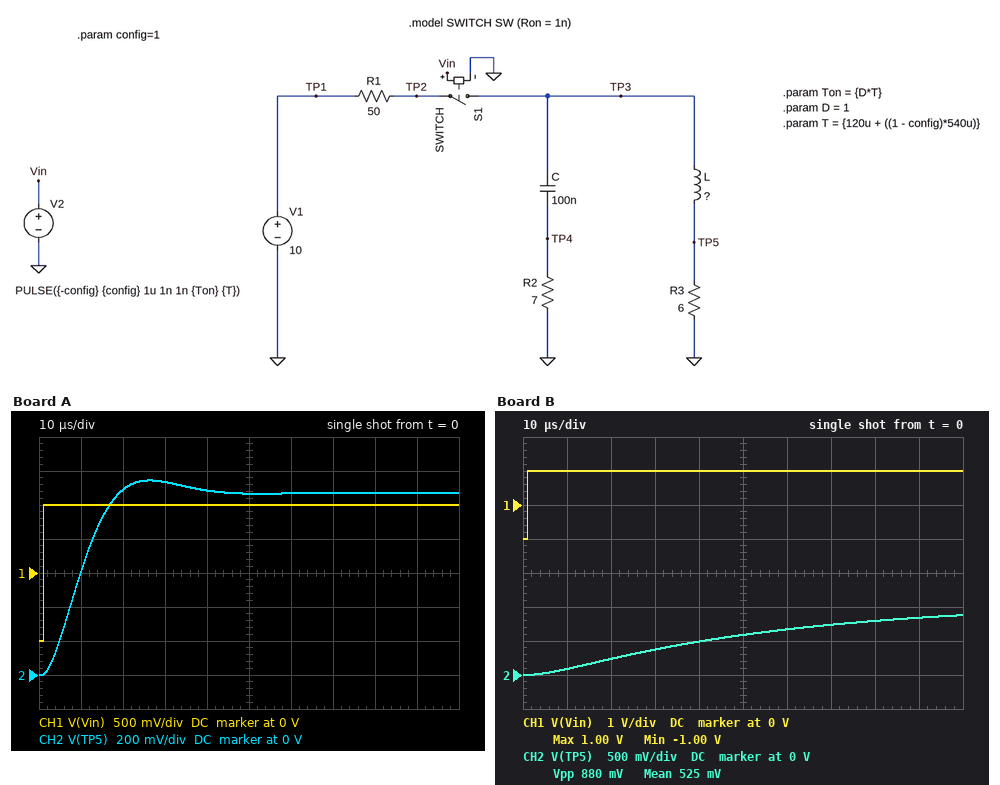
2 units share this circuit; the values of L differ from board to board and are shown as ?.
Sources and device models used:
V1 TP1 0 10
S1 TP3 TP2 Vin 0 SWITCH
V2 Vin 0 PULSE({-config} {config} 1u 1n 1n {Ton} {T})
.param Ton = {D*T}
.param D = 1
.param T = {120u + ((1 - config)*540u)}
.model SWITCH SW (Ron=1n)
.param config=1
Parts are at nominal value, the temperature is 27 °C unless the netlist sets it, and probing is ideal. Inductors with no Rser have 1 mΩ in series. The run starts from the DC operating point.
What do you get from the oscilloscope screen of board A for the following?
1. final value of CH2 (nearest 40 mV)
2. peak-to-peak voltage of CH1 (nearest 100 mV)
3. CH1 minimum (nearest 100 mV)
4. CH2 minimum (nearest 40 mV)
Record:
1.08 V
2.0 V
-1.0 V
0 V
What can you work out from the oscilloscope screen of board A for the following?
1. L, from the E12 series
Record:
390 µH
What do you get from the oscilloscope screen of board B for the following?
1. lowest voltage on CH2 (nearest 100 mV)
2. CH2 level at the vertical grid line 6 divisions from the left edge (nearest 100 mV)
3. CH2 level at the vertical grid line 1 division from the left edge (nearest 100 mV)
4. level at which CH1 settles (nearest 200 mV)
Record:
0 V
700 mV
100 mV
1.0 V
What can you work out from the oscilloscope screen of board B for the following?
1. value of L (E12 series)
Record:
3.3 mH
